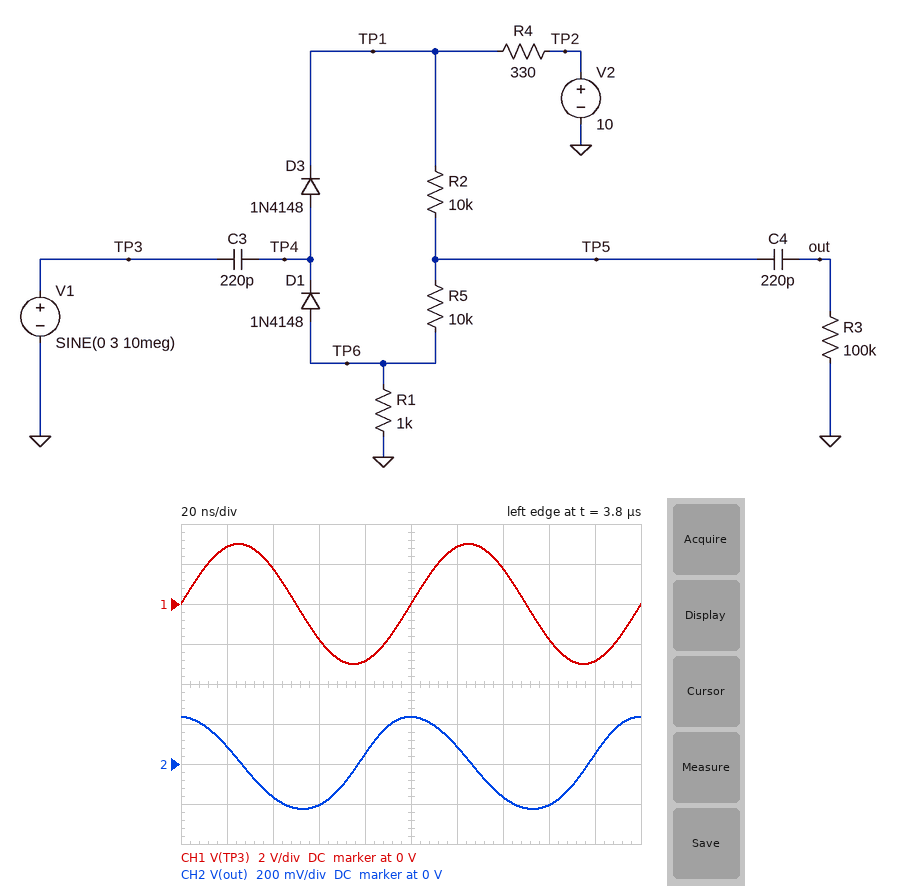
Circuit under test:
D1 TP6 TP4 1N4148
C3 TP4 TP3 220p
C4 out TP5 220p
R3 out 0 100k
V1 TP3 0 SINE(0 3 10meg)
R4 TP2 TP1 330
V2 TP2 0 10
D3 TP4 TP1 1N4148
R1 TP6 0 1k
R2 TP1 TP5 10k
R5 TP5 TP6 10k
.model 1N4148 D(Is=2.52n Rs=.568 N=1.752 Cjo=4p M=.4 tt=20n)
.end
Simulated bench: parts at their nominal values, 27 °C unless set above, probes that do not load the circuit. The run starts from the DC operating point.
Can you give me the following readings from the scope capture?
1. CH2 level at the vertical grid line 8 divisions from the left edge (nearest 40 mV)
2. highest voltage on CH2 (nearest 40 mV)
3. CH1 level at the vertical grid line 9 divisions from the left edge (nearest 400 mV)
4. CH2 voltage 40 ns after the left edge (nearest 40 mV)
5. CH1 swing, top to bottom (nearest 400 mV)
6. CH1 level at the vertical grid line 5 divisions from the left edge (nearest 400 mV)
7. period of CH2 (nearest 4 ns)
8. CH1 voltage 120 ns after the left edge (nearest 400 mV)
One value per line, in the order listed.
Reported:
-200 mV
240 mV
-2.8 V
-160 mV
6.0 V
0 V
100 ns
2.8 V
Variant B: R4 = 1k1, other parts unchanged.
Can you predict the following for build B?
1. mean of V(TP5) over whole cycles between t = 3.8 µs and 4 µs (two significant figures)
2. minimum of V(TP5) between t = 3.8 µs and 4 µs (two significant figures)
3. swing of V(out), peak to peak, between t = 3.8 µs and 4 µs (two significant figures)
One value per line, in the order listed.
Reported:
5.0 V
4.6 V
740 mV
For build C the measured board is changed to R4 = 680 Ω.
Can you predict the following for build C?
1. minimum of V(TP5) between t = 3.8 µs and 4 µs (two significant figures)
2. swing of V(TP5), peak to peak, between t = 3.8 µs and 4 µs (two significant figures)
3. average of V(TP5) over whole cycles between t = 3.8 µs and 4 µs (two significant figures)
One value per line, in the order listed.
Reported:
4.8 V
590 mV
5.1 V
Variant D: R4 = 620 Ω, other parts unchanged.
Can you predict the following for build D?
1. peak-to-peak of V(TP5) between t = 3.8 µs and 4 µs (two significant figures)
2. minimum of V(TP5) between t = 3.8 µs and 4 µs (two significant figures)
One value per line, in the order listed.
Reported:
570 mV
4.8 V
